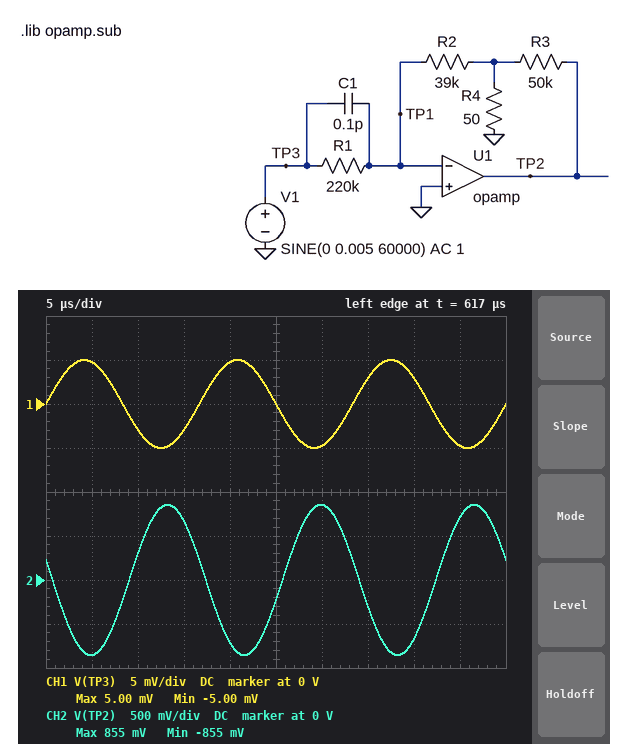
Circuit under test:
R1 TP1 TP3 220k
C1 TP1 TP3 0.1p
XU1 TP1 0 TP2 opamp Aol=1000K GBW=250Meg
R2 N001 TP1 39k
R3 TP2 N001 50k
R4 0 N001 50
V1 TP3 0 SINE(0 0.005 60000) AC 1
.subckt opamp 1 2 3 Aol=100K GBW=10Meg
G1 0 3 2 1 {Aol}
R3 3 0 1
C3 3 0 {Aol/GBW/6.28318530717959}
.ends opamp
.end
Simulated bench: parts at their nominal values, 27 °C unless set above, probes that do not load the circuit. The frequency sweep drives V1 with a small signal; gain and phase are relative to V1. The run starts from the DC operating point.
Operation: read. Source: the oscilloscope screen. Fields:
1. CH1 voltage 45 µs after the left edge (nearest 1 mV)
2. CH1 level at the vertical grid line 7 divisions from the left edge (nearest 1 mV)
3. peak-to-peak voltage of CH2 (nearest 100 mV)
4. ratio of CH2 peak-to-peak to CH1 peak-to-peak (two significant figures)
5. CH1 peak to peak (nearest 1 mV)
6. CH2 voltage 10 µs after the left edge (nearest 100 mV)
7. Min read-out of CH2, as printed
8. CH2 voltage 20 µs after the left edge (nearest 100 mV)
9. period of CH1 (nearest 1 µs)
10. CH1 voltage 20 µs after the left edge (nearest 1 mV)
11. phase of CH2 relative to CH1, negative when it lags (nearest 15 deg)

-5 mV
3 mV
1.7 V
170
10 mV
300 mV
-855 mV
-700 mV
17 µs
5 mV
165 deg
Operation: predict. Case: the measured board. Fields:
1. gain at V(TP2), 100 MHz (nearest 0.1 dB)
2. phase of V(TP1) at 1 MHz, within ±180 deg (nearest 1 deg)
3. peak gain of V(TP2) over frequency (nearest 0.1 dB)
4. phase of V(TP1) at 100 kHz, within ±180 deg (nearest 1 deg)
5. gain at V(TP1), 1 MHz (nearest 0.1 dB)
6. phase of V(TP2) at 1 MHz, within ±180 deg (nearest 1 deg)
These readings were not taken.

7.1 dB
19 deg
45.0 dB
65 deg
-16.5 dB
109 deg
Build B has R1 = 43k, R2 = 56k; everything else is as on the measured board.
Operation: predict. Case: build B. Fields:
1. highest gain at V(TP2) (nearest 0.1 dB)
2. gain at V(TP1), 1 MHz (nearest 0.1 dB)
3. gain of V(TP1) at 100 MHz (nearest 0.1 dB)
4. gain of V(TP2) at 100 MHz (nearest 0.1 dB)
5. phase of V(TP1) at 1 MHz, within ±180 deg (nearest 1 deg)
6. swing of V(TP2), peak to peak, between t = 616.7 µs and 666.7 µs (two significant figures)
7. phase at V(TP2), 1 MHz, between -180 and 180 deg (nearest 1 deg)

62.3 dB
-5.0 dB
-1.0 dB
7.0 dB
7 deg
11 V
97 deg
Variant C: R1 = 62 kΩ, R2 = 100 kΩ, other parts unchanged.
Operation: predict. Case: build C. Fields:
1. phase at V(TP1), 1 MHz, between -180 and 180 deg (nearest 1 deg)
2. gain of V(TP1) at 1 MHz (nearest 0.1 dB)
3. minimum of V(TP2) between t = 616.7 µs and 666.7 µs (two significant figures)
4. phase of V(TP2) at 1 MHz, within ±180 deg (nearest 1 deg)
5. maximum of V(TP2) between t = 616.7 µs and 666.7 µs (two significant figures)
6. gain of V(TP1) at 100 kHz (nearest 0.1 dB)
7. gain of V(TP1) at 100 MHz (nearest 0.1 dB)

6 deg
-4.2 dB
-6.8 V
96 deg
6.8 V
-7.0 dB
-0.4 dB
